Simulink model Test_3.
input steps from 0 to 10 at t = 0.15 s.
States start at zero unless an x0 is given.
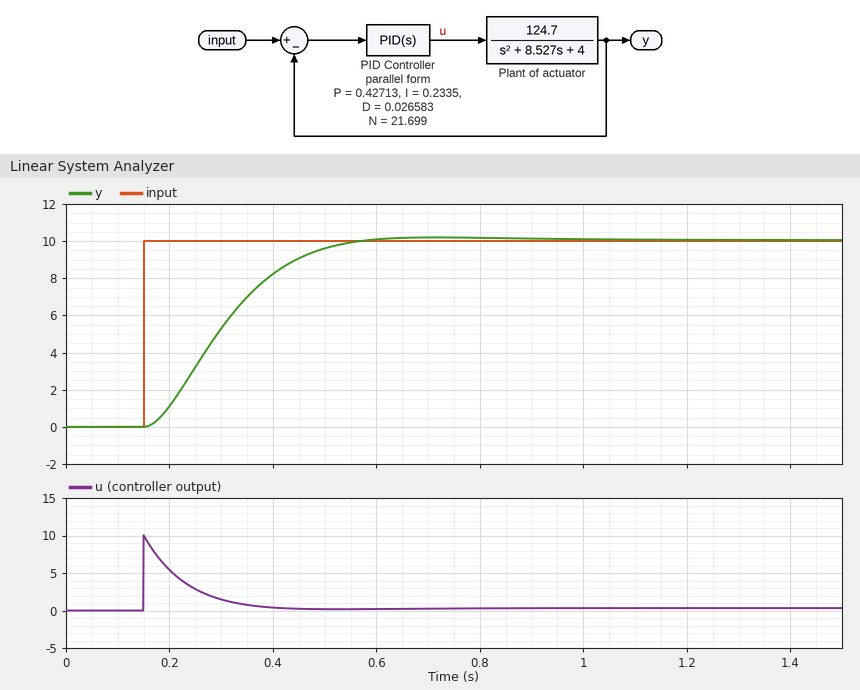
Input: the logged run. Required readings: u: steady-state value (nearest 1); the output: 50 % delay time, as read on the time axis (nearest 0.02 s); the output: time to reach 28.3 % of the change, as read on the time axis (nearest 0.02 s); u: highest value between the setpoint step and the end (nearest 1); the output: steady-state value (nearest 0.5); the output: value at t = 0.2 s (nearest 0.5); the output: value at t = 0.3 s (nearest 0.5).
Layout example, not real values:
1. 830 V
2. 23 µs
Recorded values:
1. 0
2. 0.30 s
3. 0.24 s
4. 10
5. 10.0
6. 1.0
7. 5.5
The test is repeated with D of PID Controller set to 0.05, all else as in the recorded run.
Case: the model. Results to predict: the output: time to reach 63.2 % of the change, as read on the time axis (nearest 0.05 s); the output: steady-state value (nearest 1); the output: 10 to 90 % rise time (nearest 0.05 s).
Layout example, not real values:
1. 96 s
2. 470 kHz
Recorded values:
1. 0.30 s
2. 10
3. 0.25 s
